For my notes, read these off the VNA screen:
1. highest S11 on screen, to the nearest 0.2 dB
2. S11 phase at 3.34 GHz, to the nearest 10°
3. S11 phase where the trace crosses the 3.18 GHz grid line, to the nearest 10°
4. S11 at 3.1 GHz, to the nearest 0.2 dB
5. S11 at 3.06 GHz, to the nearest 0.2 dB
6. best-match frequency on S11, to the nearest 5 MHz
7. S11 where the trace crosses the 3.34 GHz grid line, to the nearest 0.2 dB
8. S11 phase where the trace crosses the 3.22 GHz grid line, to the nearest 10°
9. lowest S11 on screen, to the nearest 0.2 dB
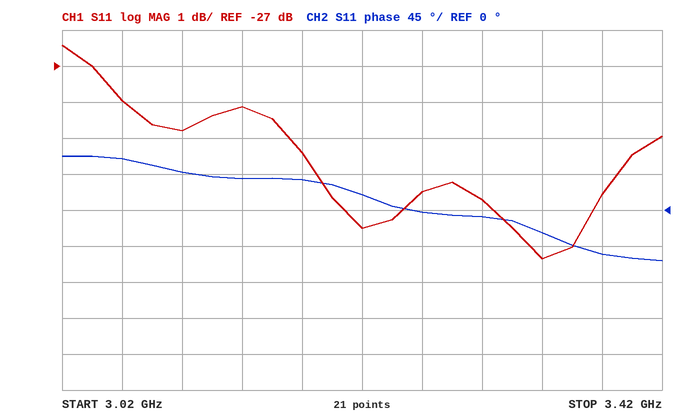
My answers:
-26.4 dB
-30°
40°
-28.8 dB
-28.0 dB
3.340 GHz
-32.4 dB
20°
-32.4 dB
